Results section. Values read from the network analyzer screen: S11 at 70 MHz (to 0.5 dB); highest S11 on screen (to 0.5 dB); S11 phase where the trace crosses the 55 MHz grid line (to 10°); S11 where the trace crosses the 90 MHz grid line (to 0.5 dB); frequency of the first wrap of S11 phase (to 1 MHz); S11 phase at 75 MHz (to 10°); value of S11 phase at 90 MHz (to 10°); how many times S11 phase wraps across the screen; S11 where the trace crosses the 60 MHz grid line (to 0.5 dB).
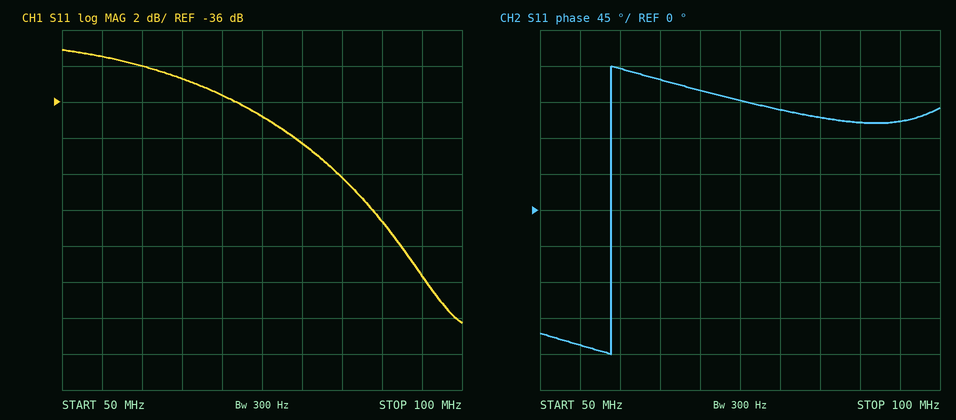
-35.5 dB
-33.0 dB
-170°
-42.5 dB
59 MHz
140°
110°
1
-34.0 dB
